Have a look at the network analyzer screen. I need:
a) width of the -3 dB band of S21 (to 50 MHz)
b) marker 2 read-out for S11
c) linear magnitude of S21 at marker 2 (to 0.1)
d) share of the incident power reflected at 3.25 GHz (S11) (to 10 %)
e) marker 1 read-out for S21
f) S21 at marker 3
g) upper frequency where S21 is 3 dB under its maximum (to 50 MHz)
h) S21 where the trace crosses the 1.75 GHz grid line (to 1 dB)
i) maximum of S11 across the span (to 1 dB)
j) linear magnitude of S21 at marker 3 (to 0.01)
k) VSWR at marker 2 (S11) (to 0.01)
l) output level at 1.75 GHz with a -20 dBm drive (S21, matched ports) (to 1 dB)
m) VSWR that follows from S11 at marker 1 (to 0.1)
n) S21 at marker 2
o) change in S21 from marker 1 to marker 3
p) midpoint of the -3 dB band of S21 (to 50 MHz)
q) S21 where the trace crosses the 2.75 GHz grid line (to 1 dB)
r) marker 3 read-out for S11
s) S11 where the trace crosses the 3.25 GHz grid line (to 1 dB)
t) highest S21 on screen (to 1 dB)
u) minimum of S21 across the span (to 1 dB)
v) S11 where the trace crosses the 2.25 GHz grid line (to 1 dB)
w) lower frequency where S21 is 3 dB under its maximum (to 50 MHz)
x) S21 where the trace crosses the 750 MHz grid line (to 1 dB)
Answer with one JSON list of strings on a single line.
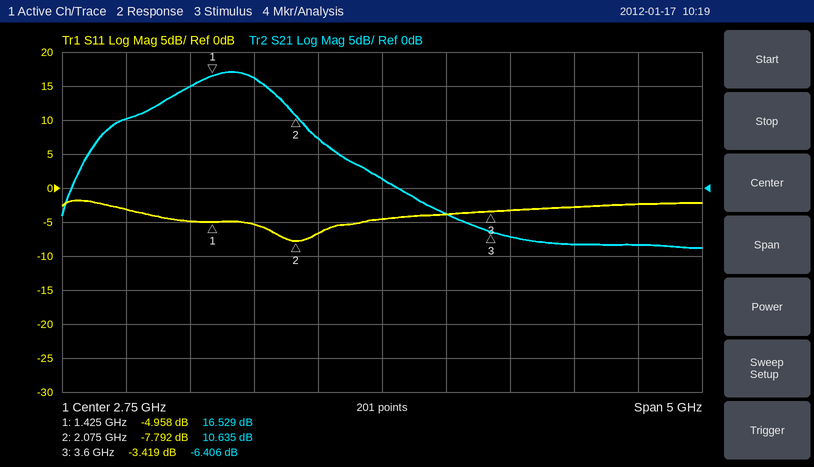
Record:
["750 MHz", "-7.792 dB", "3.4", "40 %", "16.529 dB", "-6.406 dB", "1.90 GHz", "16 dB", "-2 dB", "0.48", "2.38", "-4 dBm", "3.6", "10.635 dB", "-22.935 dB", "1.55 GHz", "1 dB", "-3.419 dB", "-4 dB", "17 dB", "-9 dB", "-7 dB", "1.15 GHz", "10 dB"]
